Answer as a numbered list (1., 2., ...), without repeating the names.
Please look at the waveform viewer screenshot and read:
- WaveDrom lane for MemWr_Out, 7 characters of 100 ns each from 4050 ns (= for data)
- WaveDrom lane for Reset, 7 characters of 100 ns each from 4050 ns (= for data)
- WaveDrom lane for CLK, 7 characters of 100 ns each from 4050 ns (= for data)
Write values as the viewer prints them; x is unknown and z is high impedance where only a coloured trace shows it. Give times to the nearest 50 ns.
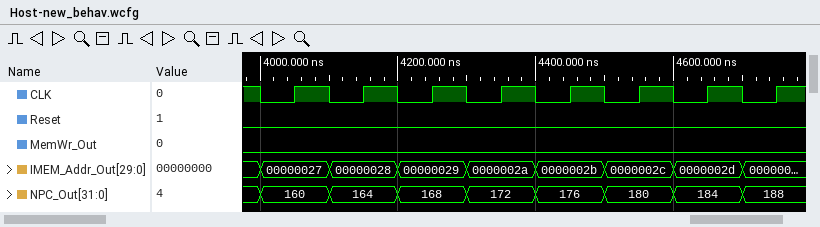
1. {name: 'MemWr_Out', wave: '0......'}
2. {name: 'Reset', wave: '0......'}
3. {name: 'CLK', wave: 'p......'}
